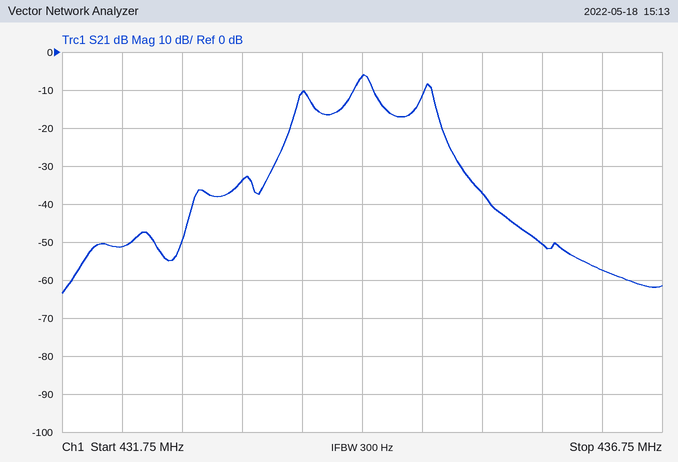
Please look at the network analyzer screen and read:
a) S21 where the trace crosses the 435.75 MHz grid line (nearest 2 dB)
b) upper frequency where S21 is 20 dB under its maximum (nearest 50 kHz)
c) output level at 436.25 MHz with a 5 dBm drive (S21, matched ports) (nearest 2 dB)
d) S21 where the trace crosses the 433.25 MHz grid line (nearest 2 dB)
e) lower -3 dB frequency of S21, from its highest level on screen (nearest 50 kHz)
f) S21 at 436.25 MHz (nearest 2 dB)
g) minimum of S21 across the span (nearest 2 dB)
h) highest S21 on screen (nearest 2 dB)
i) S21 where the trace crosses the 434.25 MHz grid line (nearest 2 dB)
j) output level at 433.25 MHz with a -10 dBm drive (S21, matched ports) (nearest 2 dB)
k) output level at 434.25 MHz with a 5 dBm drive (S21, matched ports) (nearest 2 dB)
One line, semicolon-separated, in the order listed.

-50 dB; 435.00 MHz; -52 dBm; -34 dB; 434.20 MHz; -58 dB; -64 dB; -6 dB; -6 dB; -44 dBm; -2 dBm
